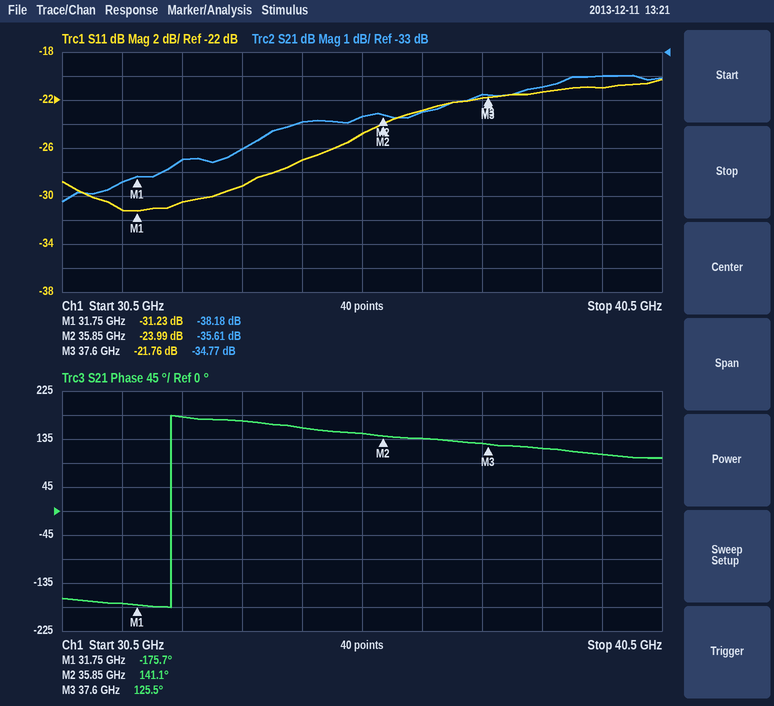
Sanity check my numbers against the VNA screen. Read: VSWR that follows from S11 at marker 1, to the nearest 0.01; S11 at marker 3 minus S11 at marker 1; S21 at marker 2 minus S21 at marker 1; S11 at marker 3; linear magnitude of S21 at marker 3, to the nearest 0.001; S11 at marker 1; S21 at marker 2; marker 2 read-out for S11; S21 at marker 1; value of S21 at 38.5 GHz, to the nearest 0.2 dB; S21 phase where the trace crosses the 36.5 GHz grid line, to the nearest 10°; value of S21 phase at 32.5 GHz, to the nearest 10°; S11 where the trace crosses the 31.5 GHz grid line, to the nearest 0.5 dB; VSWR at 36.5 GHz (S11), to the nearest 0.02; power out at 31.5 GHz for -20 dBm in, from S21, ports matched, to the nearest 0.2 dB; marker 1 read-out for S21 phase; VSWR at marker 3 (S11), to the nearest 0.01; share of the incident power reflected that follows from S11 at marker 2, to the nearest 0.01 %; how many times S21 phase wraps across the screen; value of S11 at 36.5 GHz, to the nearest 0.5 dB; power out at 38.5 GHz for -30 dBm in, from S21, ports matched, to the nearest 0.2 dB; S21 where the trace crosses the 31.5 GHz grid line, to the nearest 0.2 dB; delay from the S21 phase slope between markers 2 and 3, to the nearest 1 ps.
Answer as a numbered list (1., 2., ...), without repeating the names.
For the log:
1. 1.06
2. 9.47 dB
3. 2.57 dB
4. -21.76 dB
5. 0.018
6. -31.23 dB
7. -35.61 dB
8. -23.99 dB
9. -38.18 dB
10. -34.4 dB
11. 140°
12. 180°
13. -31.0 dB
14. 1.16
15. -58.4 dBm
16. -175.7°
17. 1.18
18. 0.40 %
19. 1
20. -23.0 dB
21. -64.4 dBm
22. -38.4 dB
23. 25 ps
